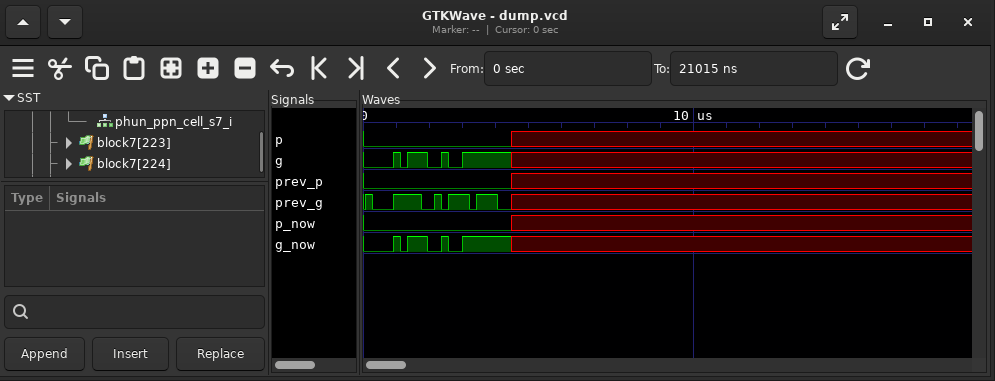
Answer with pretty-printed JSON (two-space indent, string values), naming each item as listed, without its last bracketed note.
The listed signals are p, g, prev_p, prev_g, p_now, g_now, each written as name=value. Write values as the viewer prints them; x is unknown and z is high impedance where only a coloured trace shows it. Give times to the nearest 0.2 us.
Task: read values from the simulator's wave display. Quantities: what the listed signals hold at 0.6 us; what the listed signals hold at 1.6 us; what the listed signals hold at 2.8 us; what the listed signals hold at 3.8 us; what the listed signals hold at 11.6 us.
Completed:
{
  "what the listed signals hold at 0.6 us": "p=0, g=0, prev_p=0, prev_g=0, p_now=0, g_now=0",
  "what the listed signals hold at 1.6 us": "p=0, g=1, prev_p=0, prev_g=1, p_now=0, g_now=1",
  "what the listed signals hold at 2.8 us": "p=0, g=0, prev_p=0, prev_g=1, p_now=0, g_now=0",
  "what the listed signals hold at 3.8 us": "p=0, g=1, prev_p=0, prev_g=1, p_now=0, g_now=1",
  "what the listed signals hold at 11.6 us": "p=x, g=x, prev_p=x, prev_g=x, p_now=x, g_now=x"
}
